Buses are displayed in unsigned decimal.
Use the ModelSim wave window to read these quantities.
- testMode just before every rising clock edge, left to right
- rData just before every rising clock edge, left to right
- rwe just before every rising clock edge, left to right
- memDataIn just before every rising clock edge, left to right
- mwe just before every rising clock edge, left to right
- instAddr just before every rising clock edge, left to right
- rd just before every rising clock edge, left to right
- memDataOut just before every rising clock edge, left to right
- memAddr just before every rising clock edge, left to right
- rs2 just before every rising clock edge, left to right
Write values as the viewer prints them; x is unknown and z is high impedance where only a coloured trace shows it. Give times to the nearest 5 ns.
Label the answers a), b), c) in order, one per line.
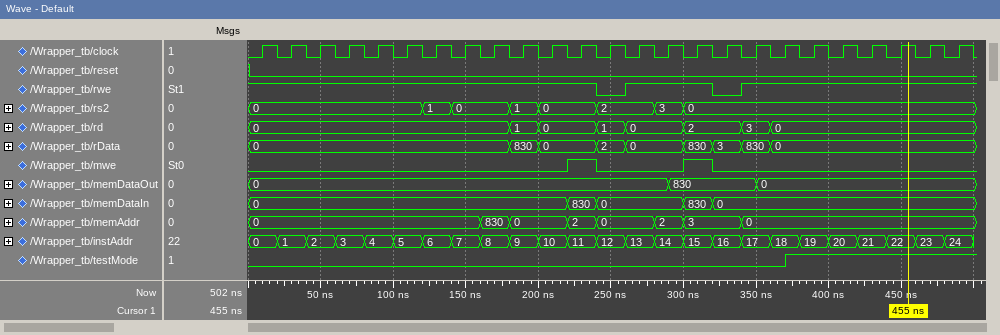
a) 0 0 0 0 0 0 0 0 0 0 0 0 0 0 0 0 0 0 0 1 1 1 1 1 1
b) 0, 0, 0, 0, 0, 0, 0, 0, 0, 830, 0, 0, 2, 0, 0, 830, 3, 830, 0, 0, 0, 0, 0, 0, 0
c) 1 1 1 1 1 1 1 1 1 1 1 1 0 1 1 1 0 1 1 1 1 1 1 1 1
d) 0, 0, 0, 0, 0, 0, 0, 0, 0, 0, 0, 830, 0, 0, 0, 830, 0, 0, 0, 0, 0, 0, 0, 0, 0
e) 0 0 0 0 0 0 0 0 0 0 0 1 0 0 0 1 0 0 0 0 0 0 0 0 0
f) 0, 1, 2, 3, 4, 5, 6, 7, 8, 9, 10, 11, 12, 13, 14, 15, 16, 17, 18, 19, 20, 21, 22, 23, 24
g) 0, 0, 0, 0, 0, 0, 0, 0, 0, 1, 0, 0, 1, 0, 0, 2, 2, 3, 0, 0, 0, 0, 0, 0, 0
h) 0, 0, 0, 0, 0, 0, 0, 0, 0, 0, 0, 0, 0, 0, 0, 830, 830, 830, 0, 0, 0, 0, 0, 0, 0
i) 0, 0, 0, 0, 0, 0, 0, 0, 830, 0, 0, 2, 0, 0, 2, 3, 3, 0, 0, 0, 0, 0, 0, 0, 0
j) 0, 0, 0, 0, 0, 0, 1, 0, 0, 1, 0, 0, 2, 2, 3, 0, 0, 0, 0, 0, 0, 0, 0, 0, 0
